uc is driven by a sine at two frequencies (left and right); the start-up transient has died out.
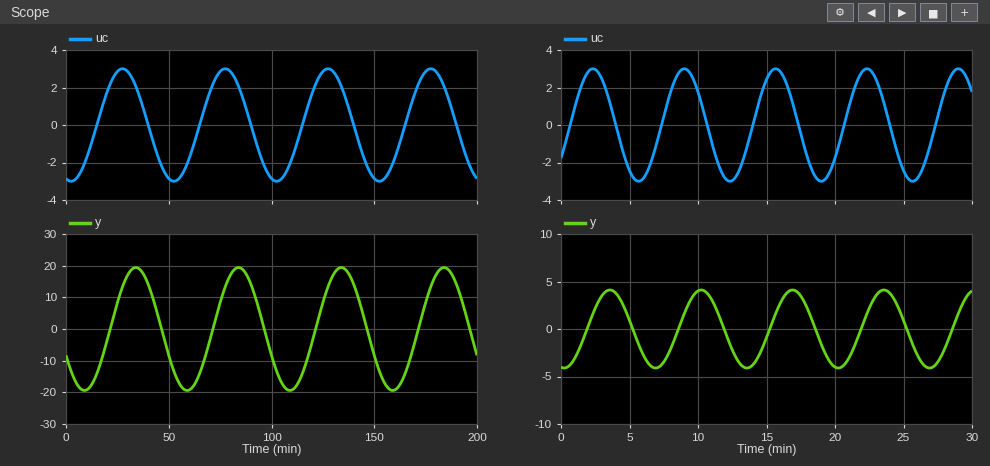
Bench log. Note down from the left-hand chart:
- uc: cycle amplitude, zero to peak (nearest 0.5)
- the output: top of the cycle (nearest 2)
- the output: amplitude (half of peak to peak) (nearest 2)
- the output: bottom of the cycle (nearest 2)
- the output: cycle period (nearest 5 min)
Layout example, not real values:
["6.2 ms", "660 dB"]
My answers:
["3.0", "20", "20", "-20", "50 min"]
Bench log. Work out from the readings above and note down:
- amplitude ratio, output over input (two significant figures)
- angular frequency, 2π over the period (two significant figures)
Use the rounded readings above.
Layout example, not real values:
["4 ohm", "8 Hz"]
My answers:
["6.7", "0.13 rad/min"]
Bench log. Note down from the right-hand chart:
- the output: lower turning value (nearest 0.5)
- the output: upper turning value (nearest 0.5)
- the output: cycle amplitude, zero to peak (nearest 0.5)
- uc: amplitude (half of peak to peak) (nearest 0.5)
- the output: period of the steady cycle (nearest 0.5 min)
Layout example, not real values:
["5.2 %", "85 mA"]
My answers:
["-4.0", "4.0", "4.0", "3.0", "6.5 min"]
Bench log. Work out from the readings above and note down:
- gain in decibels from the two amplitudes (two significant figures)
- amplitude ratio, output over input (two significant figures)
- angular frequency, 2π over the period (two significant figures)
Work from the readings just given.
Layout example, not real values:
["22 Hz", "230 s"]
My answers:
["2.5 dB", "1.3", "0.97 rad/min"]
